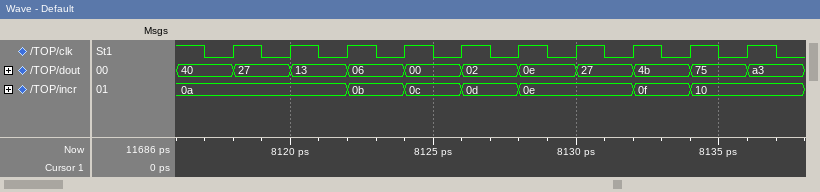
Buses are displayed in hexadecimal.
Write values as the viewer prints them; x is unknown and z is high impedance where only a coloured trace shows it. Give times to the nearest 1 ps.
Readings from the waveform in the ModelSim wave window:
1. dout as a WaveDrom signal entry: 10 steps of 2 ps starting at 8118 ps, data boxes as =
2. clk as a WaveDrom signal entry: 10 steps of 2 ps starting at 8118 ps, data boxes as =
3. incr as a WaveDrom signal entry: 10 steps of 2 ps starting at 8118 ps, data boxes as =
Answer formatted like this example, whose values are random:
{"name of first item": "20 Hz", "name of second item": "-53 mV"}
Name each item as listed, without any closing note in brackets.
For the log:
{"dout as a WaveDrom signal entry: 10 steps of 2 ps starting at 8118 ps, data boxes as =": "{name: 'dout', wave: '==========', data: '27 13 06 00 02 0e 27 4b 75 a3'}", "clk as a WaveDrom signal entry: 10 steps of 2 ps starting at 8118 ps, data boxes as =": "{name: 'clk', wave: 'p.........'}", "incr as a WaveDrom signal entry: 10 steps of 2 ps starting at 8118 ps, data boxes as =": "{name: 'incr', wave: '=.====.==.', data: '0a 0b 0c 0d 0e 0f 10'}"}
